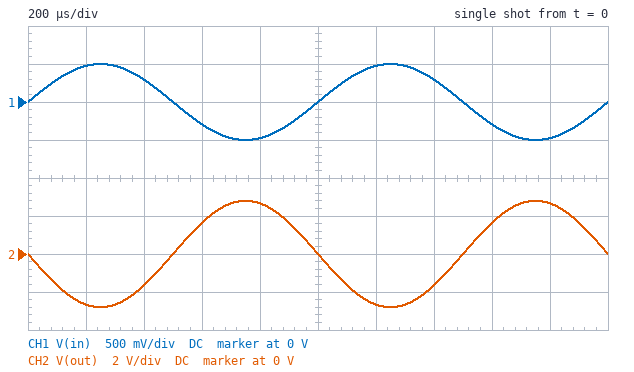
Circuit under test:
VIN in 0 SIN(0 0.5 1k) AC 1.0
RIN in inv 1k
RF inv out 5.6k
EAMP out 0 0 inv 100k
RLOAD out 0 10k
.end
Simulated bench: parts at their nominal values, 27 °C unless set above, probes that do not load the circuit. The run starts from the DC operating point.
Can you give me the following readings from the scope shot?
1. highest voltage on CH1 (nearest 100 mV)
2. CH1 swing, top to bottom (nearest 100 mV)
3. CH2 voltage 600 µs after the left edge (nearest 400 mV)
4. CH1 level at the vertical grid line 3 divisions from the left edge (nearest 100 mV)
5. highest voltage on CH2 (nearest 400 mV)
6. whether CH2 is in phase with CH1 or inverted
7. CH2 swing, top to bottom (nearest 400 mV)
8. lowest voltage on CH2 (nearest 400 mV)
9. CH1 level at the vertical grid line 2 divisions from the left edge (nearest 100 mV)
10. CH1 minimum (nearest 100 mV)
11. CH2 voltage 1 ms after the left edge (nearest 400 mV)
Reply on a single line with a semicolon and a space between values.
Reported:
500 mV; 1.0 V; 1.6 V; -300 mV; 2.8 V; inverted; 5.6 V; -2.8 V; 300 mV; -500 mV; 0 V
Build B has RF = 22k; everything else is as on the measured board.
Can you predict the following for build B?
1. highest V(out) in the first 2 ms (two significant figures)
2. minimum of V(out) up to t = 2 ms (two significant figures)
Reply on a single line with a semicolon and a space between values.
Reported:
11 V; -11 V
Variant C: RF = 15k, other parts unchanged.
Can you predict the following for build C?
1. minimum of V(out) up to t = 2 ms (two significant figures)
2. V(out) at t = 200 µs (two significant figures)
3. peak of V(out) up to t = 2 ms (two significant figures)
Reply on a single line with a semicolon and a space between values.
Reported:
-7.5 V; -7.1 V; 7.5 V
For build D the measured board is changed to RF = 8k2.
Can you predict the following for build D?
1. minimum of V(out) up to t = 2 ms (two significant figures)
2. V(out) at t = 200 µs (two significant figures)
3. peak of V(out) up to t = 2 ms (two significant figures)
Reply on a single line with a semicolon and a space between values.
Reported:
-4.1 V; -3.9 V; 4.1 V
